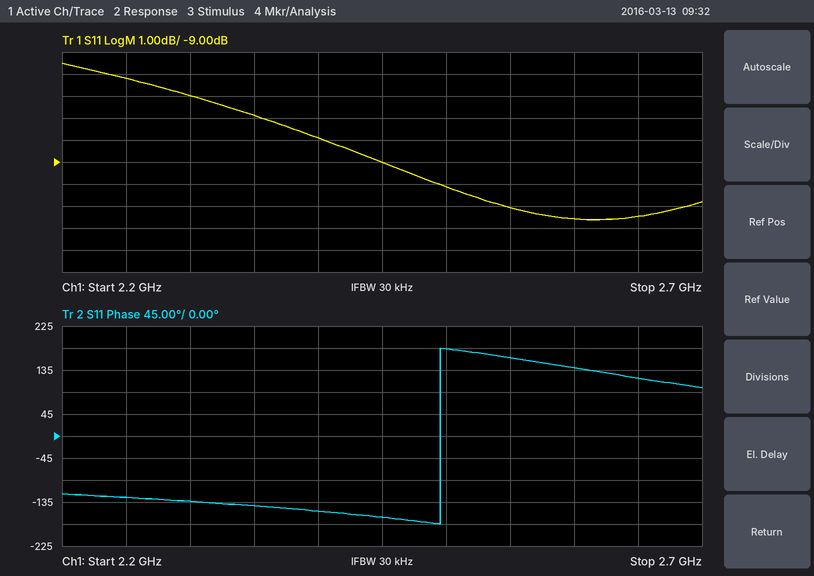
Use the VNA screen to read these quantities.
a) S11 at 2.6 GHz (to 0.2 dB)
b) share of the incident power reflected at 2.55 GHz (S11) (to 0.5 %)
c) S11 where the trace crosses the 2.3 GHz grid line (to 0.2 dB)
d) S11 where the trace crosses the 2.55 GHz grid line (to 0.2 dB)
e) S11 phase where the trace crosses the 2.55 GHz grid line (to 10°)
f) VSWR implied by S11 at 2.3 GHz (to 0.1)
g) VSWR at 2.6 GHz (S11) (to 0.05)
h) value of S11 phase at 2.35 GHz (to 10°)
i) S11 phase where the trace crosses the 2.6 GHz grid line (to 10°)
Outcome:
-11.6 dB
8.0 %
-6.0 dB
-11.0 dB
160°
3.0
1.70
-140°
140°
